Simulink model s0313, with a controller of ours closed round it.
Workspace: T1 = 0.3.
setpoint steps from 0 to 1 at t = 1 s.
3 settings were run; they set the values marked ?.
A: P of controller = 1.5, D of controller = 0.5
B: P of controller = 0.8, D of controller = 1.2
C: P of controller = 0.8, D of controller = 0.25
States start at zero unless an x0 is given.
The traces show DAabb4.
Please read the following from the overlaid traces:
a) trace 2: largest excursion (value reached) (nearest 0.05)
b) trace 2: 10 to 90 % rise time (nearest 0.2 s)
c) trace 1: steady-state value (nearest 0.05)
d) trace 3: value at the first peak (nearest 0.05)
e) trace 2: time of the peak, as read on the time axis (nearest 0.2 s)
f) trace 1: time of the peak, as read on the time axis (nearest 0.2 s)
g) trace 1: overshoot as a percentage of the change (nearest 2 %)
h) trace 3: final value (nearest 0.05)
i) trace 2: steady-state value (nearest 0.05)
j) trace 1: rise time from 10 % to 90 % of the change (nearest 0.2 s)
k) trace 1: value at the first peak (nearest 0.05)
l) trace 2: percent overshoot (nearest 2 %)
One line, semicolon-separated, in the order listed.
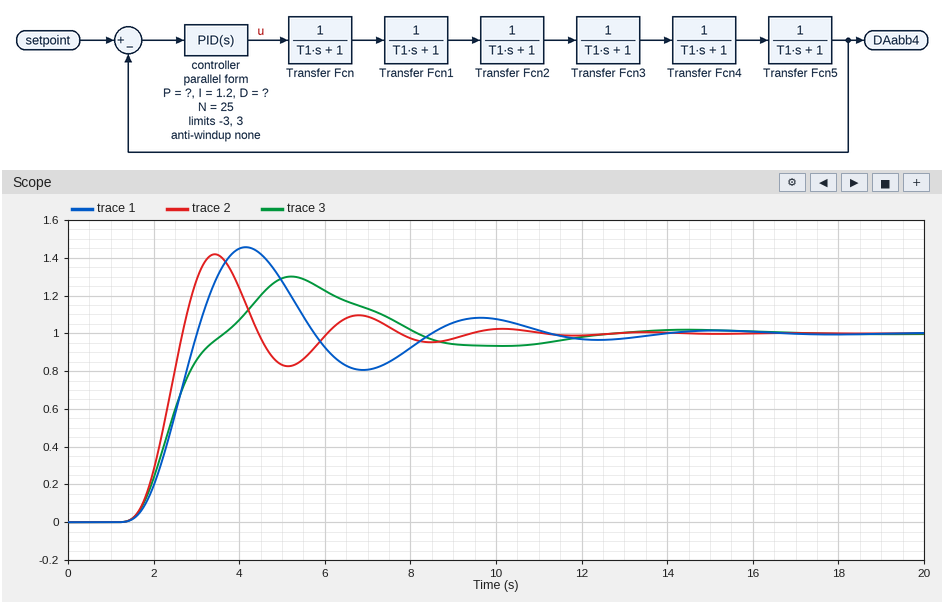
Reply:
1.40; 0.8 s; 1.00; 1.30; 3.4 s; 4.2 s; 46 %; 1.00; 1.00; 1.0 s; 1.45; 42 %
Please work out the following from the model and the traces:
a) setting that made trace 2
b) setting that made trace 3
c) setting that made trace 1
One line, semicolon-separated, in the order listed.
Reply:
A; B; C
